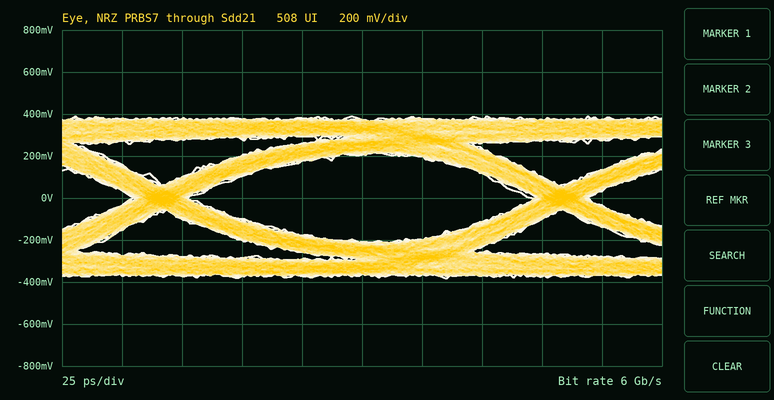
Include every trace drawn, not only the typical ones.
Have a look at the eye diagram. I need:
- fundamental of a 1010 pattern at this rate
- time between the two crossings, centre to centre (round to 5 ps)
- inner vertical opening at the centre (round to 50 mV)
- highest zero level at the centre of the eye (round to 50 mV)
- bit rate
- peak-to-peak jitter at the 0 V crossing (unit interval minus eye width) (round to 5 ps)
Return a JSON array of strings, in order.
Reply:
["3 GHz", "165 ps", "400 mV", "-200 mV", "6 Gb/s", "25 ps"]
